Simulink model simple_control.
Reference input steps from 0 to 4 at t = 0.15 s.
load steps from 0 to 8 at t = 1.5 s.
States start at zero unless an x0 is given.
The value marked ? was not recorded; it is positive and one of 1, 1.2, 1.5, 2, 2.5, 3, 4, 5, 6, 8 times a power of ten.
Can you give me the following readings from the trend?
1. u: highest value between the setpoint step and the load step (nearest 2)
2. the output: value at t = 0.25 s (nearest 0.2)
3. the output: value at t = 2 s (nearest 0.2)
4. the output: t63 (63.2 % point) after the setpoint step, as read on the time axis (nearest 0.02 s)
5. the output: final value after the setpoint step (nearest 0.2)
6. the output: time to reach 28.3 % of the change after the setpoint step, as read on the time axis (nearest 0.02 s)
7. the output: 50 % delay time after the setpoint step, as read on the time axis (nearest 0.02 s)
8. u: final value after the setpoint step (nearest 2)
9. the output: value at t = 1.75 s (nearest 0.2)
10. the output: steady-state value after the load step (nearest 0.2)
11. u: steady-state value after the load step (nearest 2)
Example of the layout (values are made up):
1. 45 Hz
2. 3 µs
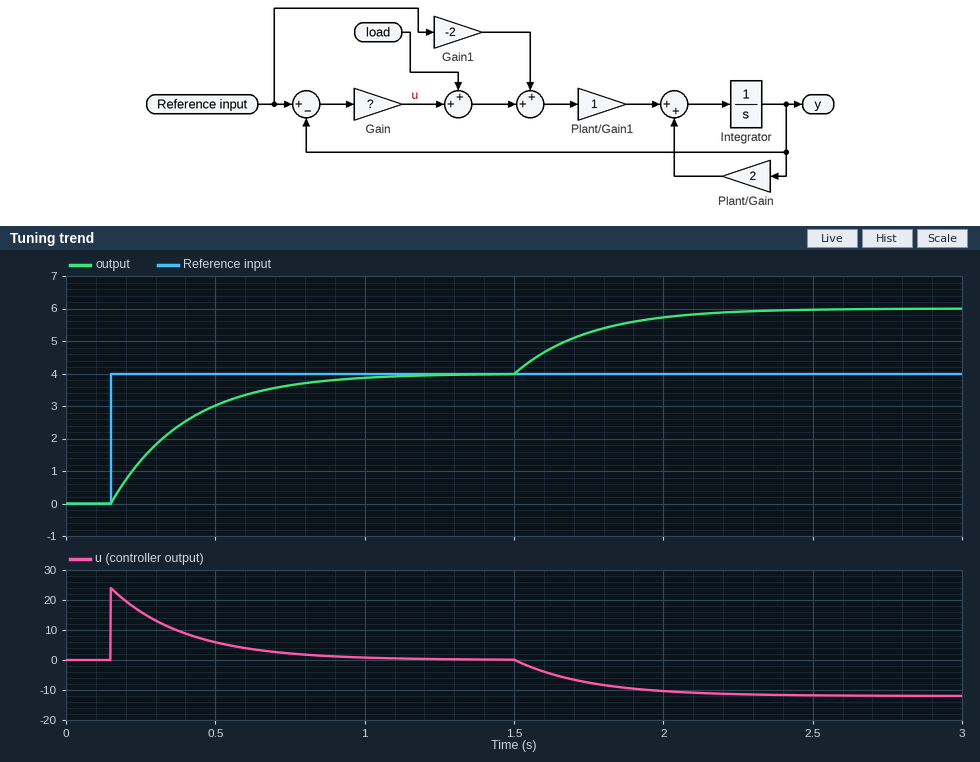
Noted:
1. 24
2. 1.4
3. 5.8
4. 0.40 s
5. 4.0
6. 0.24 s
7. 0.32 s
8. 0
9. 5.2
10. 6.0
11. -12
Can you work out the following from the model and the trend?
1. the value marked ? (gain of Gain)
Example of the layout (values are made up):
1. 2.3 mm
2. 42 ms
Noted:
1. 6
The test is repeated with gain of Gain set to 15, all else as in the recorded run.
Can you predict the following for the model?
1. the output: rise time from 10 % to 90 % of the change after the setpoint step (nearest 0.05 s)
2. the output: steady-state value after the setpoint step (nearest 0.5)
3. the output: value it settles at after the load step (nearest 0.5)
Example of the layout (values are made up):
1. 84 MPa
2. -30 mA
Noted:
1. 0.15 s
2. 4.0
3. 4.5
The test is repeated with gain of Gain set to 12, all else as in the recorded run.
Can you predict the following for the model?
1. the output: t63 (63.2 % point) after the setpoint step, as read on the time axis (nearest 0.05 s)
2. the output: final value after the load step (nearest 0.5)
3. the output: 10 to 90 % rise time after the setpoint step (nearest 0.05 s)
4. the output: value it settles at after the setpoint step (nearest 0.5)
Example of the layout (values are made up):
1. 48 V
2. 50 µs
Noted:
1. 0.25 s
2. 5.0
3. 0.20 s
4. 4.0
